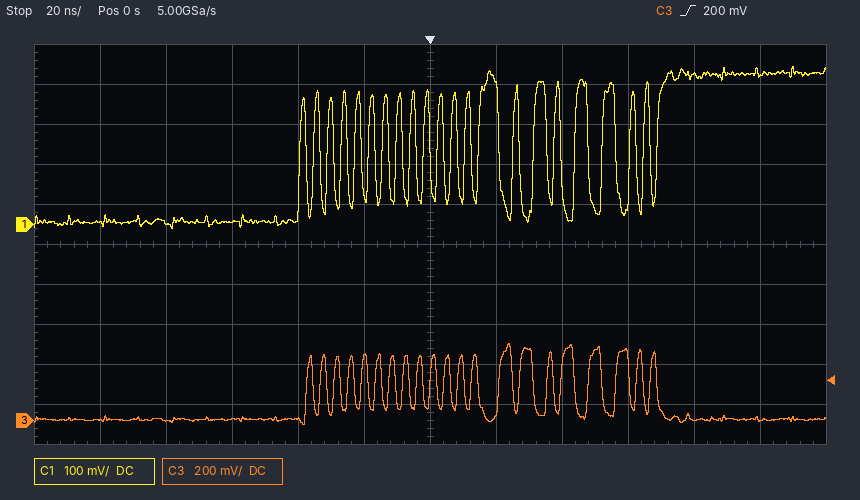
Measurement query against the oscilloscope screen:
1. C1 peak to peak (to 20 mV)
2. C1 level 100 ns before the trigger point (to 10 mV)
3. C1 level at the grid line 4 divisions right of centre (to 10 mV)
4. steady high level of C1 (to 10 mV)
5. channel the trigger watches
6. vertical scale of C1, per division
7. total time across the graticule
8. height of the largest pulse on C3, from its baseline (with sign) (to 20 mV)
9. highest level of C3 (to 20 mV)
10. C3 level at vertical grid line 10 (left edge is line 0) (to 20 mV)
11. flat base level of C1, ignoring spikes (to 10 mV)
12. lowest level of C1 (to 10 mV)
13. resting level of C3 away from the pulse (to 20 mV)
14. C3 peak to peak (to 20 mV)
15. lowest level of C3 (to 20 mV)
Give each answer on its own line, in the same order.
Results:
400 mV
0 mV
370 mV
380 mV
C3
100 mV
240 ns
+380 mV
380 mV
0 mV
10 mV
-10 mV
0 mV
400 mV
-20 mV
